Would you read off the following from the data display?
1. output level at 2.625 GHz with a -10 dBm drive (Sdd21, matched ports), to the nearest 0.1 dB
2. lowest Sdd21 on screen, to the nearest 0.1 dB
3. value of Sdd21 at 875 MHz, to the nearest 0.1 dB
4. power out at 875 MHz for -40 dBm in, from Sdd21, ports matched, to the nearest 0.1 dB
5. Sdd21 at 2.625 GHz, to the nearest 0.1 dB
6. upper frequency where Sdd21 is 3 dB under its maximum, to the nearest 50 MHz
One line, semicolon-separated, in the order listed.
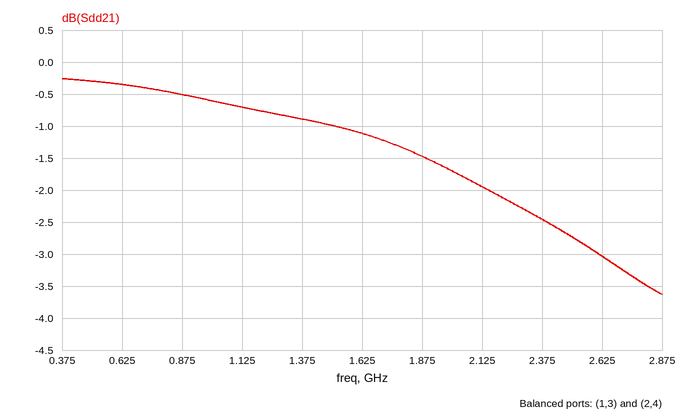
-13.0 dBm; -3.6 dB; -0.5 dB; -40.5 dBm; -3.0 dB; 2.70 GHz
